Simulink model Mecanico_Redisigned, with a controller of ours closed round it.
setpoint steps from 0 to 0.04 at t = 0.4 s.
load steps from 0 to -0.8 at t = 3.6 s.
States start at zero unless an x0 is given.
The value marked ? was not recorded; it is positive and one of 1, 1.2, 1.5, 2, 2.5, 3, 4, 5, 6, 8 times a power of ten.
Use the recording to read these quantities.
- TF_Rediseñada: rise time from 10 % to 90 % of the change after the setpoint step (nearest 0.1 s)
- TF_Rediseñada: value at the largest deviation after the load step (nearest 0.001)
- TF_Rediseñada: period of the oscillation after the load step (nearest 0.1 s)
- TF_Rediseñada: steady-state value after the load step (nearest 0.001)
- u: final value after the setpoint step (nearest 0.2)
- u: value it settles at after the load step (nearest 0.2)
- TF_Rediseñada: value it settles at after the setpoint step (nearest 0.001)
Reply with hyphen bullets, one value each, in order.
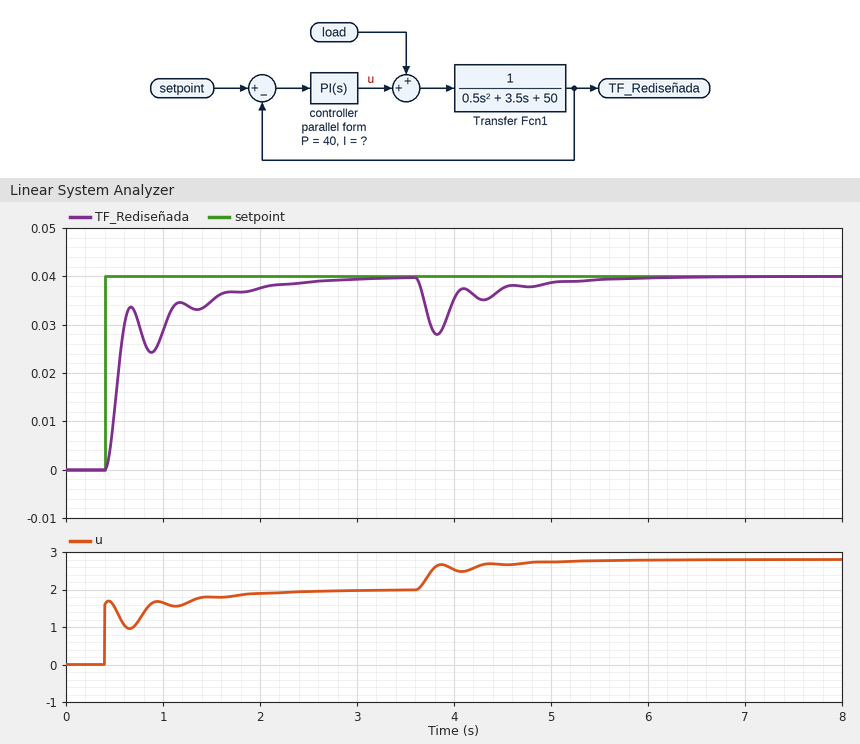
- 1.1 s
- 0.028
- 0.5 s
- 0.040
- 2.0
- 2.8
- 0.040
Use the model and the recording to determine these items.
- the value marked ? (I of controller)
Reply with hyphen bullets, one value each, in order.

- 120
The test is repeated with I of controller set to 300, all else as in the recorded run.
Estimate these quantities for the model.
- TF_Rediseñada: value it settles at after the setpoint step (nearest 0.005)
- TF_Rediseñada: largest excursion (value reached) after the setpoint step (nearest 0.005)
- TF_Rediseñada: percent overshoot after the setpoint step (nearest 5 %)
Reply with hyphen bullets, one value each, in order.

- 0.040
- 0.045
- 15 %
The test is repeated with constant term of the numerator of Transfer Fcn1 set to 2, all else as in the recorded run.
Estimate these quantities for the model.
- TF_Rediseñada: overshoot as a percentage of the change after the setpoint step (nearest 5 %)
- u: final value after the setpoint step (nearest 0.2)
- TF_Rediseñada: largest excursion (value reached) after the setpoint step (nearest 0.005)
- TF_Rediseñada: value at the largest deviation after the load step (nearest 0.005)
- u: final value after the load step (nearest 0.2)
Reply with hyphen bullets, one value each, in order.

- 15 %
- 1.0
- 0.045
- 0.025
- 1.8
